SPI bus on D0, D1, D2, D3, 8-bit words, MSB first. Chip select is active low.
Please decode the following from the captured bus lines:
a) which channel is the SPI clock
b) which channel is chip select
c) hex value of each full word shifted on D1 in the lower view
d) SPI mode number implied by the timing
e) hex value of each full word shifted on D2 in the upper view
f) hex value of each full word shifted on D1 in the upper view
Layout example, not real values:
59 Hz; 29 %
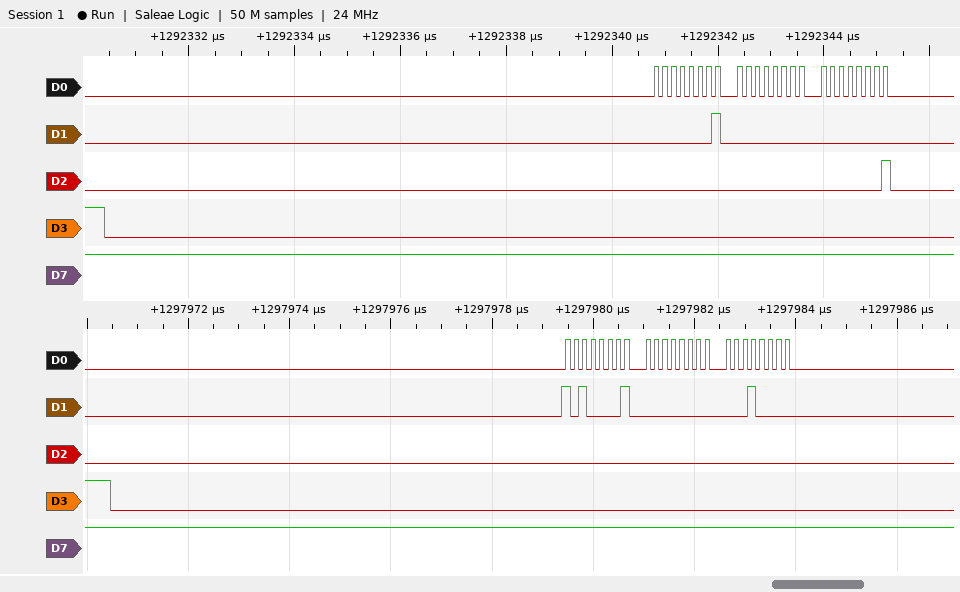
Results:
D0; D3; A1, 00, 10; 0; 00, 00, 01; 01, 00, 00
